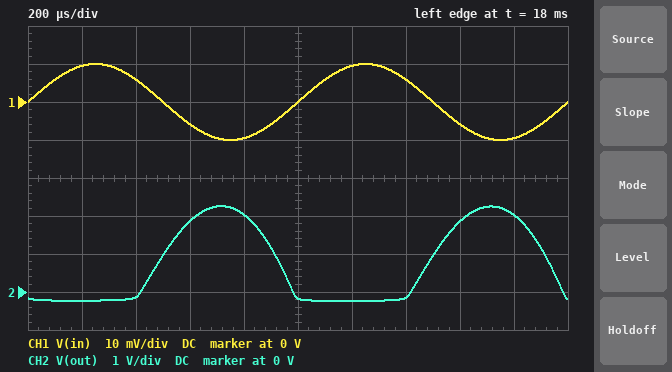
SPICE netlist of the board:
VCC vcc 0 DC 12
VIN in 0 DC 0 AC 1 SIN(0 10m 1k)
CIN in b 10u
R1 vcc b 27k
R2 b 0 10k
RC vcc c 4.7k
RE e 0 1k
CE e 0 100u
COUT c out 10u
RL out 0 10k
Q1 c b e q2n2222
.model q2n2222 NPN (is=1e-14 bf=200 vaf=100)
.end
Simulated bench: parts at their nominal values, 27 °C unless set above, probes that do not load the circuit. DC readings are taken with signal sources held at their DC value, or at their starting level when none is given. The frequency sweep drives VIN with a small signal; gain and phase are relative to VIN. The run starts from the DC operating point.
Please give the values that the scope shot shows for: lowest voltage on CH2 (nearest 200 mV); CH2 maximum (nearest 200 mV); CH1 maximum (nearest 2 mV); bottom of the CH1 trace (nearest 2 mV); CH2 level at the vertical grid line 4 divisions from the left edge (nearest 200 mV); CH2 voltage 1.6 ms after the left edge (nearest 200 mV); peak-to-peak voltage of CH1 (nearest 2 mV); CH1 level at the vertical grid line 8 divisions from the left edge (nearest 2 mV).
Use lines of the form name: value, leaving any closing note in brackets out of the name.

lowest voltage on CH2: -200 mV
CH2 maximum: 2.2 V
CH1 maximum: 10 mV
bottom of the CH1 trace: -10 mV
CH2 level at the vertical grid line 4 divisions from the left edge: 2.0 V
CH2 voltage 1.6 ms after the left edge: 1.8 V
peak-to-peak voltage of CH1: 20 mV
CH1 level at the vertical grid line 8 divisions from the left edge: -6 mV
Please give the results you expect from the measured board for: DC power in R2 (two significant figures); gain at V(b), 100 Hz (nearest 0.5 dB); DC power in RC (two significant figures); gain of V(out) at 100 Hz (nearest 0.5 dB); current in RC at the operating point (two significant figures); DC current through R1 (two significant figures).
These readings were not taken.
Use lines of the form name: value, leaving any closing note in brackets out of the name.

DC power in R2: 790 µW
gain at V(b), 100 Hz: -15.0 dB
DC power in RC: 20 mW
gain of V(out) at 100 Hz: 9.0 dB
current in RC at the operating point: 2.1 mA
DC current through R1: 340 µA
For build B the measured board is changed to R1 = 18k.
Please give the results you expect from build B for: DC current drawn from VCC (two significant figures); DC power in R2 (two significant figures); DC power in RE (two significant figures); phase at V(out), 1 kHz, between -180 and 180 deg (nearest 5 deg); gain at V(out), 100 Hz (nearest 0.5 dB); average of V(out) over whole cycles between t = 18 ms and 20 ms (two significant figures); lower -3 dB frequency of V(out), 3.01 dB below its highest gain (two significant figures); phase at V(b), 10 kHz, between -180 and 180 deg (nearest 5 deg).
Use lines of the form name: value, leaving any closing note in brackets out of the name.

DC current drawn from VCC: 2.6 mA
DC power in R2: 870 µW
DC power in RE: 5.1 mW
phase at V(out), 1 kHz, between -180 and 180 deg: -140 deg
gain at V(out), 100 Hz: -4.0 dB
average of V(out) over whole cycles between t = 18 ms and 20 ms: 230 mV
lower -3 dB frequency of V(out), 3.01 dB below its highest gain: 830 Hz
phase at V(b), 10 kHz, between -180 and 180 deg: 5 deg
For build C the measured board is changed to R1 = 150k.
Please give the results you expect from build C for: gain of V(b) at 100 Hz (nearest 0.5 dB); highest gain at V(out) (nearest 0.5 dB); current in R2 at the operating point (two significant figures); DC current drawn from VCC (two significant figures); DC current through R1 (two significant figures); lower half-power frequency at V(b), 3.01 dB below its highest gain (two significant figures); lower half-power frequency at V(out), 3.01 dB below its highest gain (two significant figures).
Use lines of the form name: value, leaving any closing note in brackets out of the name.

gain of V(b) at 100 Hz: 0 dB
highest gain at V(out): 25.0 dB
current in R2 at the operating point: 74 µA
DC current drawn from VCC: 220 µA
DC current through R1: 75 µA
lower half-power frequency at V(b), 3.01 dB below its highest gain: 1.8 Hz
lower half-power frequency at V(out), 3.01 dB below its highest gain: 11 Hz
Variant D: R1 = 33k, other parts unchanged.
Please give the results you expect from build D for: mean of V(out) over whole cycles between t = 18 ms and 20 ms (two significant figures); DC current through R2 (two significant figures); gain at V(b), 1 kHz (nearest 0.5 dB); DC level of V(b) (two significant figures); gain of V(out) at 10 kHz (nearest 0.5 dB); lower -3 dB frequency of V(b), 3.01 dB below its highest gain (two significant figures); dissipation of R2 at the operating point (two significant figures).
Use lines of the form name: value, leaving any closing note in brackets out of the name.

mean of V(out) over whole cycles between t = 18 ms and 20 ms: 840 mV
DC current through R2: 270 µA
gain at V(b), 1 kHz: 0 dB
DC level of V(b): 2.7 V
gain of V(out) at 10 kHz: 47.5 dB
lower -3 dB frequency of V(b), 3.01 dB below its highest gain: 2.3 Hz
dissipation of R2 at the operating point: 740 µW
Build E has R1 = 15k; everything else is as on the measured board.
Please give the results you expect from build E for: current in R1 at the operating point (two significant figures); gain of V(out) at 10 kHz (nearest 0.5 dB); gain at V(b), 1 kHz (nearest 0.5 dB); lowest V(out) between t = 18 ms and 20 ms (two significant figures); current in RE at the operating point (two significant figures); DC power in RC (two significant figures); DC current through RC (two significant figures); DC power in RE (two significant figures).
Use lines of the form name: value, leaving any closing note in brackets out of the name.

current in R1 at the operating point: 600 µA
gain of V(out) at 10 kHz: 11.0 dB
gain at V(b), 1 kHz: -2.5 dB
lowest V(out) between t = 18 ms and 20 ms: -35 mV
current in RE at the operating point: 2.3 mA
DC power in RC: 20 mW
DC current through RC: 2.0 mA
DC power in RE: 5.5 mW
